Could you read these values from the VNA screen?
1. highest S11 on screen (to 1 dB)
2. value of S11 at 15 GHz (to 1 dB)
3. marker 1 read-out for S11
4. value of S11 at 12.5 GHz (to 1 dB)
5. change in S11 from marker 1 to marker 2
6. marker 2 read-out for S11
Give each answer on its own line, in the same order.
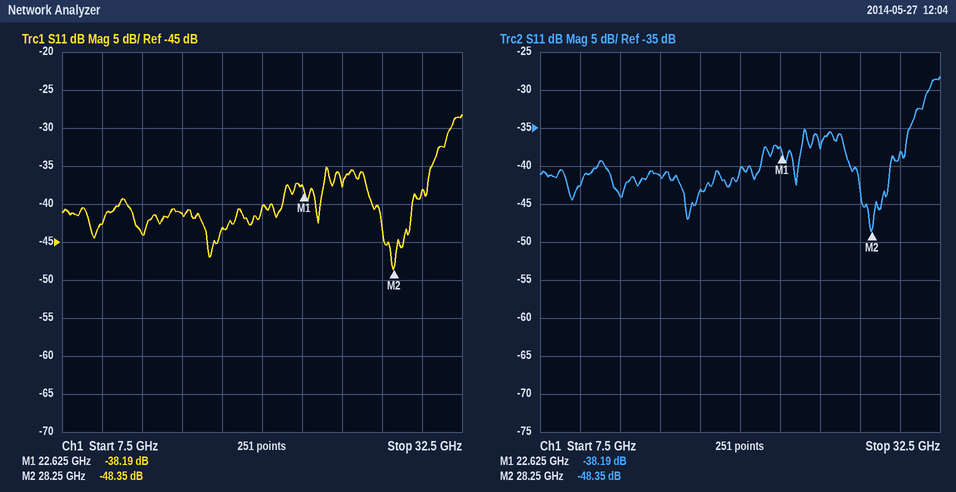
-28 dB
-41 dB
-38.19 dB
-44 dB
-10.16 dB
-48.35 dB
